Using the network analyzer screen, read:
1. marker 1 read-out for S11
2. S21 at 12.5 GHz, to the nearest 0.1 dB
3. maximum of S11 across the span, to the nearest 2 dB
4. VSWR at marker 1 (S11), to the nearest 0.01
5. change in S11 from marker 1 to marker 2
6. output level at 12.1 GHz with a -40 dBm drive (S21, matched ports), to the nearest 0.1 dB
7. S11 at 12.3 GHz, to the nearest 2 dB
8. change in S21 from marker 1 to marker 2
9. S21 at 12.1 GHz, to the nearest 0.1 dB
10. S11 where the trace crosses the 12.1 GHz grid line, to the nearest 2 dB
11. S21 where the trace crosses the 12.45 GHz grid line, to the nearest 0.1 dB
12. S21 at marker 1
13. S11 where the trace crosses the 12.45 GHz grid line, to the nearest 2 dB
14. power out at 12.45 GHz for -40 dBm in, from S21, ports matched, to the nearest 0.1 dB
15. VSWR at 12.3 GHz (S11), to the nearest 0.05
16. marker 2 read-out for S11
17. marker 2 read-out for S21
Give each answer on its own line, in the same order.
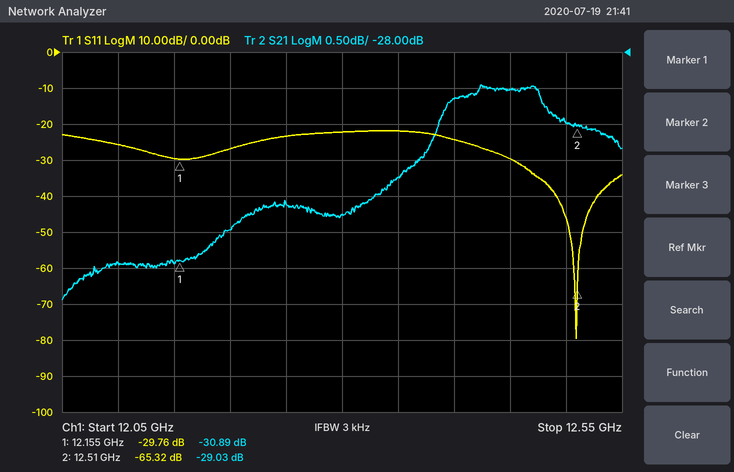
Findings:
-29.76 dB
-29.0 dB
-22 dB
1.07
-35.56 dB
-70.9 dBm
-22 dB
1.86 dB
-30.9 dB
-26 dB
-28.5 dB
-30.89 dB
-30 dB
-68.5 dBm
1.15
-65.32 dB
-29.03 dB
